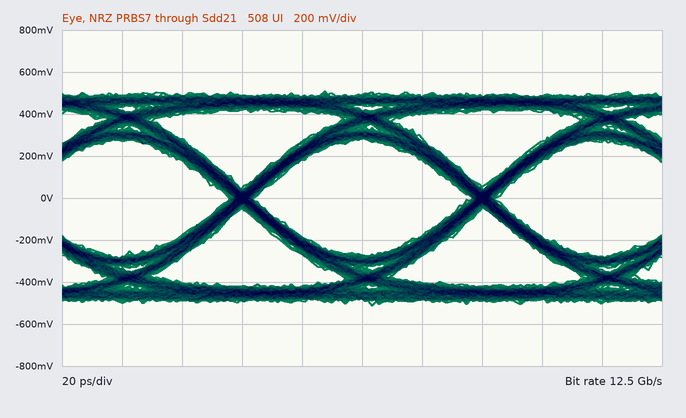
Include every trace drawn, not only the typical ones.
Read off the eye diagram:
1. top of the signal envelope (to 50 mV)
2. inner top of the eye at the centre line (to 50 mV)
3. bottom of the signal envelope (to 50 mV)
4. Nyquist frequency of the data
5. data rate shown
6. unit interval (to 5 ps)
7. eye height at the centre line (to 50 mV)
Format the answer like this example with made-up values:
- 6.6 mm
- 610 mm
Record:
- 500 mV
- 300 mV
- -500 mV
- 6.25 GHz
- 12.5 Gb/s
- 80 ps
- 550 mV
